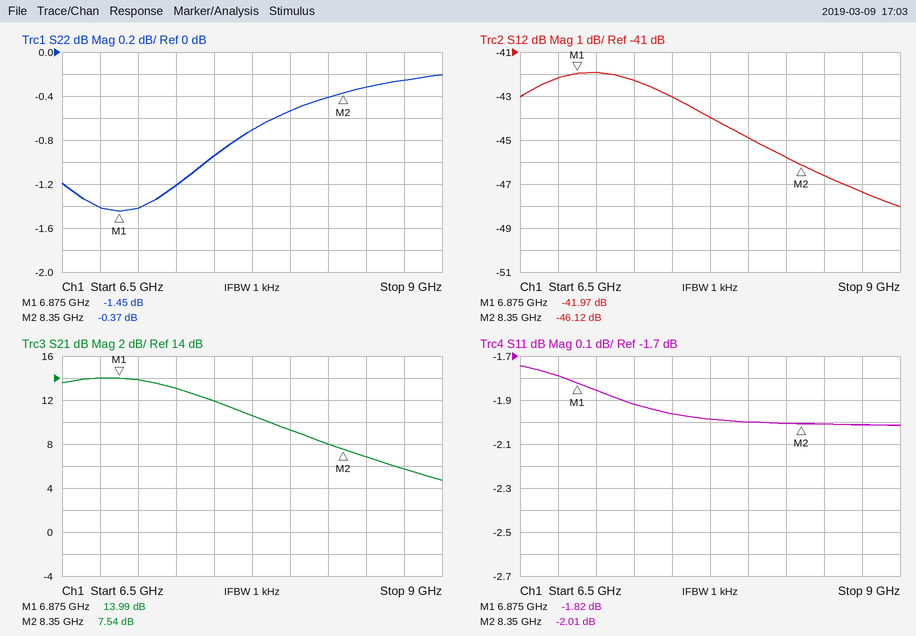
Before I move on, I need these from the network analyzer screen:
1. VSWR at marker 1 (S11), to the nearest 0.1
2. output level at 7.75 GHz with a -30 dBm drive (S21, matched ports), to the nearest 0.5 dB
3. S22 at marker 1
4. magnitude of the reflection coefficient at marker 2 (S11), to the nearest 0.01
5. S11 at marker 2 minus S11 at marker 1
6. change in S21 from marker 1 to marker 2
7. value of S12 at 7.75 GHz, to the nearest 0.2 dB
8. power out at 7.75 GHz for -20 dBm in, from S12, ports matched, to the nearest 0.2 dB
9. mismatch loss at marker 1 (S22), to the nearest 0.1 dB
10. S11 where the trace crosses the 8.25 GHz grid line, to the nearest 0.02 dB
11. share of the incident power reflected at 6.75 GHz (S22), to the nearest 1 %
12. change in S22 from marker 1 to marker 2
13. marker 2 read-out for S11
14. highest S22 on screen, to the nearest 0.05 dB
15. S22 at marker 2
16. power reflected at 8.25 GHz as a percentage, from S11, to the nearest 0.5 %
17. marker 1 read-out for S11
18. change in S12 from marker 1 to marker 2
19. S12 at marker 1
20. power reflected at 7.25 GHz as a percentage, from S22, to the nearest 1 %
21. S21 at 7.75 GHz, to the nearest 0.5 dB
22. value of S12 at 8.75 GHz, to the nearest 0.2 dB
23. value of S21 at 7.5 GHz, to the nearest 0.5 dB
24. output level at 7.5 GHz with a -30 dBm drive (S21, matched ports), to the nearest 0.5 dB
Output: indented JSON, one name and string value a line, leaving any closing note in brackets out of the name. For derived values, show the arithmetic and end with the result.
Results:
{
  "VSWR at marker 1 (S11), to the nearest 0.1": "(1 + 0.8110)/(1 − 0.8110) ≈ 9.6",
  "output level at 7.75 GHz with a -30 dBm drive (S21, matched ports), to the nearest 0.5 dB": "-30 dBm + (10.5 dB) = -19.5 dBm",
  "S22 at marker 1": "-1.45 dB",
  "magnitude of the reflection coefficient at marker 2 (S11), to the nearest 0.01": "10^(-2.01/20) ≈ 0.79",
  "S11 at marker 2 minus S11 at marker 1": "-2.01 − (-1.82) = -0.19 dB",
  "change in S21 from marker 1 to marker 2": "7.54 − (13.99) = -6.45 dB",
  "value of S12 at 7.75 GHz, to the nearest 0.2 dB": "-44.0 dB",
  "power out at 7.75 GHz for -20 dBm in, from S12, ports matched, to the nearest 0.2 dB": "-20 dBm + (-44.0 dB) = -64.0 dBm",
  "mismatch loss at marker 1 (S22), to the nearest 0.1 dB": "−10 log10(1 − 10^(-1.45/10)) ≈ 5.5 dB",
  "S11 where the trace crosses the 8.25 GHz grid line, to the nearest 0.02 dB": "-2.00 dB",
  "share of the incident power reflected at 6.75 GHz (S22), to the nearest 1 %": "10^(-1.4/10) ≈ 72 %",
  "change in S22 from marker 1 to marker 2": "-0.37 − (-1.45) = 1.08 dB",
  "marker 2 read-out for S11": "-2.01 dB",
  "highest S22 on screen, to the nearest 0.05 dB": "-0.20 dB",
  "S22 at marker 2": "-0.37 dB",
  "power reflected at 8.25 GHz as a percentage, from S11, to the nearest 0.5 %": "10^(-2/10) ≈ 63.1 %, so 63.0 % to the nearest 0.5 %",
  "marker 1 read-out for S11": "-1.82 dB",
  "change in S12 from marker 1 to marker 2": "-46.12 − (-41.97) = -4.15 dB",
  "S12 at marker 1": "-41.97 dB",
  "power reflected at 7.25 GHz as a percentage, from S22, to the nearest 1 %": "10^(-1.2/10) ≈ 76 %",
  "S21 at 7.75 GHz, to the nearest 0.5 dB": "10.5 dB",
  "value of S12 at 8.75 GHz, to the nearest 0.2 dB": "-47.4 dB",
  "value of S21 at 7.5 GHz, to the nearest 0.5 dB": "12.0 dB",
  "output level at 7.5 GHz with a -30 dBm drive (S21, matched ports), to the nearest 0.5 dB": "-30 dBm + (12.0 dB) = -18.0 dBm"
}
